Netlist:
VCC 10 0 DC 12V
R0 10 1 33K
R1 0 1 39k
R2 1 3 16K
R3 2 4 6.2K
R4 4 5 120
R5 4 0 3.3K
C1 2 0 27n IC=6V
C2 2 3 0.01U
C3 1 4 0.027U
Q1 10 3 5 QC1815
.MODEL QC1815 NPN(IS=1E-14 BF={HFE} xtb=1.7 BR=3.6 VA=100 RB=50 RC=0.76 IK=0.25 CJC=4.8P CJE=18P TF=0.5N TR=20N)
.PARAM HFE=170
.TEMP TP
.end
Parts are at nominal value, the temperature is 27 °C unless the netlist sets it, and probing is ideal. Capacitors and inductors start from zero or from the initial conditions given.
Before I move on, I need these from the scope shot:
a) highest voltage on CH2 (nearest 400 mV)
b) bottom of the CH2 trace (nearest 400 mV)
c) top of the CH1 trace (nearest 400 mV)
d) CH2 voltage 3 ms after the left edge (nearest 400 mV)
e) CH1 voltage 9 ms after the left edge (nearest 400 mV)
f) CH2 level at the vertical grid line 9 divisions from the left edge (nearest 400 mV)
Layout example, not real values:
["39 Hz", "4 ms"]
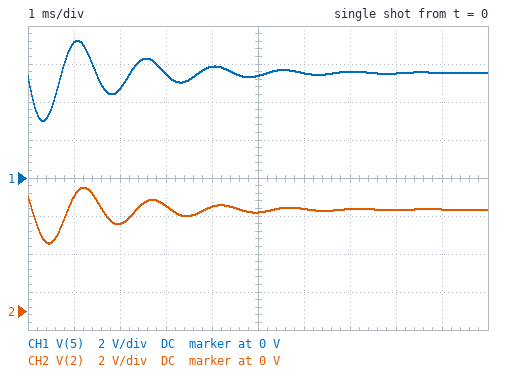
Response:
["6.4 V", "3.6 V", "7.2 V", "5.6 V", "5.6 V", "5.2 V"]
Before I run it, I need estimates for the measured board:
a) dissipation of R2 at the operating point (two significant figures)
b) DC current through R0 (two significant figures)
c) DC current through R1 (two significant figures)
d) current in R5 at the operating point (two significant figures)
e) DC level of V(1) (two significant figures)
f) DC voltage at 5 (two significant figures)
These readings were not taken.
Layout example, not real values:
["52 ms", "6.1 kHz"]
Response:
["1.3 µW", "170 µA", "160 µA", "1.6 mA", "6.3 V", "5.5 V"]
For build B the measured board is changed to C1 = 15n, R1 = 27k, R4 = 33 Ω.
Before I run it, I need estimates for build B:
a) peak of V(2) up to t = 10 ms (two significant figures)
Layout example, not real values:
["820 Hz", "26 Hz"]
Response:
["6.7 V"]
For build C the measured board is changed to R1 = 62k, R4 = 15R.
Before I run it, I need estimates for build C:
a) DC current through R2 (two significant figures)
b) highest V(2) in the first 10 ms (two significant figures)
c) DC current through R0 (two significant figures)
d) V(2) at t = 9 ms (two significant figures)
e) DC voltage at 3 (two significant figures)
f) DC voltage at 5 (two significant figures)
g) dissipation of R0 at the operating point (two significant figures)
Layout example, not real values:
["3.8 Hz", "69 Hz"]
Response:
["11 µA", "8.6 V", "130 µA", "7.1 V", "7.4 V", "6.7 V", "590 µW"]
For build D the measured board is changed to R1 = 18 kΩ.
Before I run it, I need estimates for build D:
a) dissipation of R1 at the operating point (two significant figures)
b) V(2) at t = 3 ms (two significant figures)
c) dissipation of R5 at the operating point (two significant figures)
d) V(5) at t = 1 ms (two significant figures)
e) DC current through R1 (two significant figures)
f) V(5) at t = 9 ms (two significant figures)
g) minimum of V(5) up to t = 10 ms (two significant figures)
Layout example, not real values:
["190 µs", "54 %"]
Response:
["970 µW", "3.2 V", "3.3 mW", "4.5 V", "230 µA", "3.4 V", "1.3 V"]
